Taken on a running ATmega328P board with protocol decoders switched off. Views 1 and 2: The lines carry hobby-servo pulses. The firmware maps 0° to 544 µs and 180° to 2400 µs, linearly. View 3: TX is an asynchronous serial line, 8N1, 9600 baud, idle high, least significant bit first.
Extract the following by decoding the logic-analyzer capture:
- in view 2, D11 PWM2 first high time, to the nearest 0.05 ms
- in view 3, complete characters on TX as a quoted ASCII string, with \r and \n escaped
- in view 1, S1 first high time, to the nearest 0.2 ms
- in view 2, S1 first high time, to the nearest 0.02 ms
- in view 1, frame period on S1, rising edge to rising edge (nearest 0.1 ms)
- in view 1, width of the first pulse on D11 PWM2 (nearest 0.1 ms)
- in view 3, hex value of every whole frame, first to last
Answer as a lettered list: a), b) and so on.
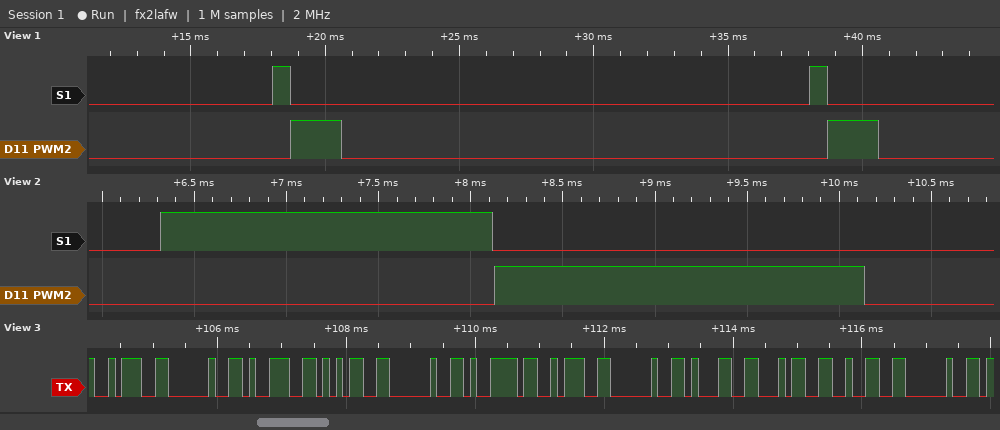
a) 2.00 ms
b) ": 95 y: 142 "
c) 0.6 ms
d) 1.80 ms
e) 20.0 ms
f) 1.9 ms
g) 3A 20 39 35 20 79 3A 20 31 34 32 20
